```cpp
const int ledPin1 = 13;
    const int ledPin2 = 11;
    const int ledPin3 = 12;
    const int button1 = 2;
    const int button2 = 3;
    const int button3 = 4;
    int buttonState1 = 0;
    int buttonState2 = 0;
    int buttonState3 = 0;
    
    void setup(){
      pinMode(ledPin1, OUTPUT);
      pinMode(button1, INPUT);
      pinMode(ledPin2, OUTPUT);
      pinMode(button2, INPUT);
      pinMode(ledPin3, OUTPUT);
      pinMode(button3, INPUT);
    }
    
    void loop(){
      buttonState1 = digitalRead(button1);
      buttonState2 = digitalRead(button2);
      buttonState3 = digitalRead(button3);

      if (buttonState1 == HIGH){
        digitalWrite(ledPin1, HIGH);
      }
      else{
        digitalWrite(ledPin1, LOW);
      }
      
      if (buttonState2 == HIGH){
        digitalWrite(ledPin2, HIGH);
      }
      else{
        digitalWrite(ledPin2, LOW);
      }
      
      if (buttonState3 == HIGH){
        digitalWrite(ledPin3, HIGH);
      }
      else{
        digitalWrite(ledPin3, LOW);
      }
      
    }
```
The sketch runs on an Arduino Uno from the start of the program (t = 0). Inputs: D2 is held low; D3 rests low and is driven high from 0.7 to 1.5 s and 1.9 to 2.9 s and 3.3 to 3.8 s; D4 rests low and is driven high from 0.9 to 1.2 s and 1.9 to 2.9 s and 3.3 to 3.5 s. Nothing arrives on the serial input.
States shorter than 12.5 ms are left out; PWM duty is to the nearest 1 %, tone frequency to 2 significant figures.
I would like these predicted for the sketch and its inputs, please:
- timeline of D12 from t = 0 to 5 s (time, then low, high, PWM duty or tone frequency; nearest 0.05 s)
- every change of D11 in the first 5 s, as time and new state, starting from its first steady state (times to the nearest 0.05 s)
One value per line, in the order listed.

0 s low; 0.9 s high; 1.2 s low; 1.9 s high; 2.9 s low; 3.3 s high; 3.5 s low
0 s low; 0.7 s high; 1.5 s low; 1.9 s high; 2.9 s low; 3.3 s high; 3.8 s low
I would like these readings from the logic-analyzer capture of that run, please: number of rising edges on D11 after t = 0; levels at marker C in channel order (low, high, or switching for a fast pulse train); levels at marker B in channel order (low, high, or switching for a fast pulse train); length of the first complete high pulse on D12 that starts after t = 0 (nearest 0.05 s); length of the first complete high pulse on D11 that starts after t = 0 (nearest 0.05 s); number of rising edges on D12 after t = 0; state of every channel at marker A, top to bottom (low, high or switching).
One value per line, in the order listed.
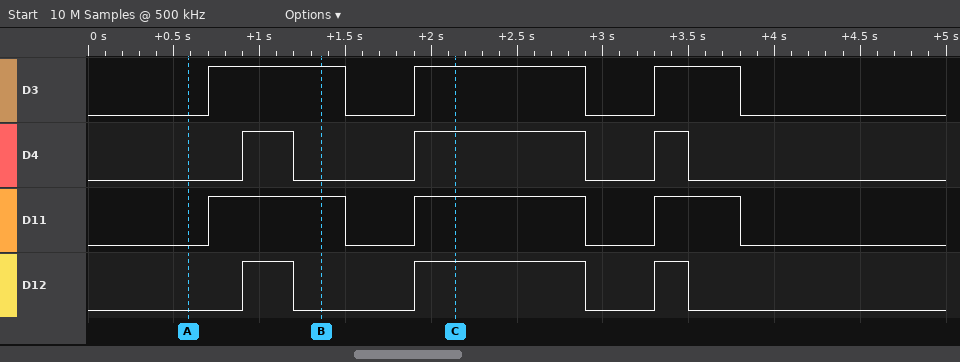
3
D3 high, D4 high, D11 high, D12 high
D3 high, D4 low, D11 high, D12 low
0.30 s
0.80 s
3
D3 low, D4 low, D11 low, D12 low
